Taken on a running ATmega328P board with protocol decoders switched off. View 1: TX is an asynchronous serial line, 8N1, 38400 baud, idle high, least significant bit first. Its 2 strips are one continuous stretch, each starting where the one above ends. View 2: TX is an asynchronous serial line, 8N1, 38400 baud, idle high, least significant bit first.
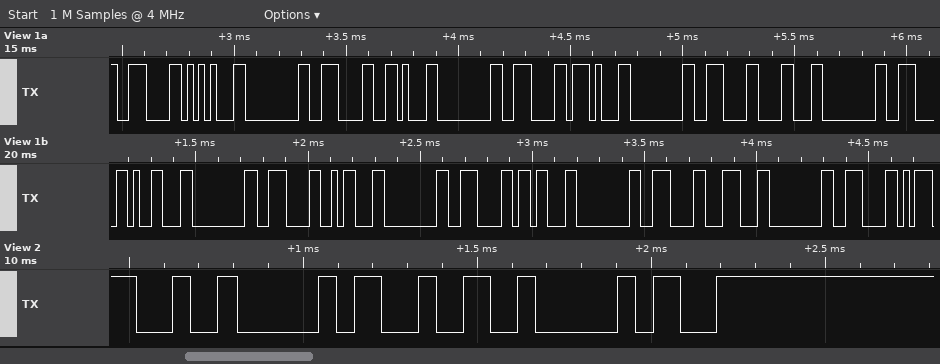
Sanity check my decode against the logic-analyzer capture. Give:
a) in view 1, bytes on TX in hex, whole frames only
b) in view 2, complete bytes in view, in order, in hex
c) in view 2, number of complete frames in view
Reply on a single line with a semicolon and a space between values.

0E 15 00 0E 16 00 0E 17 00 0E 18 00 0E 19 00 0E 1A 00 0E 1B 00 0E 1C 00 0E; 18 00 0E 1C 00 0E; 6
